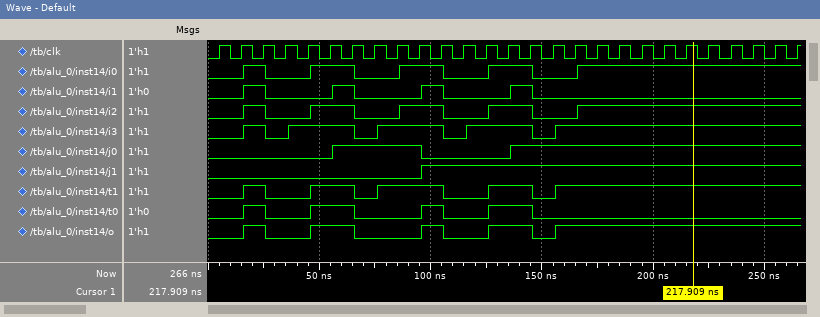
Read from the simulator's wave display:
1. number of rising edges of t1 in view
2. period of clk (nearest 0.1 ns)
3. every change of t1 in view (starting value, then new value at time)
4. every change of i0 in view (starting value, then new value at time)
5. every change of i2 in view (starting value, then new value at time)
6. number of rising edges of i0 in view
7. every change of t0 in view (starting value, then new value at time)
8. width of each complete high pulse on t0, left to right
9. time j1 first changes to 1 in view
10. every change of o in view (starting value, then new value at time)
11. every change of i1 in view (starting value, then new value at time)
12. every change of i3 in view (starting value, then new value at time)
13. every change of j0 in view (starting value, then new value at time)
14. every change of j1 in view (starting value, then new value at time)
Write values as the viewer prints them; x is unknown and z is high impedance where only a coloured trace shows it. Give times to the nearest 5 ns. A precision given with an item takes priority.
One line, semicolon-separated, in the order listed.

5; 10 ns; 0, 1 at 15 ns, 0 at 25 ns, 1 at 45 ns, 0 at 65 ns, 1 at 75 ns, 0 at 105 ns, 1 at 125 ns, 0 at 145 ns, 1 at 155 ns; 0, 1 at 15 ns, 0 at 25 ns, 1 at 45 ns, 0 at 65 ns, 1 at 85 ns, 0 at 105 ns, 1 at 125 ns, 0 at 145 ns, 1 at 165 ns; 0, 1 at 15 ns, 0 at 25 ns, 1 at 45 ns, 0 at 65 ns, 1 at 85 ns, 0 at 105 ns, 1 at 125 ns, 0 at 145 ns, 1 at 165 ns; 5; 0, 1 at 15 ns, 0 at 25 ns, 1 at 45 ns, 0 at 65 ns, 1 at 95 ns, 0 at 105 ns, 1 at 125 ns, 0 at 145 ns; 10 ns, 20 ns, 10 ns, 20 ns; 95 ns; 0, 1 at 15 ns, 0 at 25 ns, 1 at 45 ns, 0 at 65 ns, 1 at 95 ns, 0 at 105 ns, 1 at 125 ns, 0 at 145 ns, 1 at 155 ns; 0, 1 at 15 ns, 0 at 25 ns, 1 at 55 ns, 0 at 65 ns, 1 at 95 ns, 0 at 105 ns, 1 at 135 ns, 0 at 145 ns; 0, 1 at 15 ns, 0 at 25 ns, 1 at 35 ns, 0 at 65 ns, 1 at 75 ns, 0 at 105 ns, 1 at 115 ns, 0 at 145 ns, 1 at 155 ns; 0, 1 at 55 ns, 0 at 95 ns, 1 at 135 ns; 0, 1 at 95 ns
